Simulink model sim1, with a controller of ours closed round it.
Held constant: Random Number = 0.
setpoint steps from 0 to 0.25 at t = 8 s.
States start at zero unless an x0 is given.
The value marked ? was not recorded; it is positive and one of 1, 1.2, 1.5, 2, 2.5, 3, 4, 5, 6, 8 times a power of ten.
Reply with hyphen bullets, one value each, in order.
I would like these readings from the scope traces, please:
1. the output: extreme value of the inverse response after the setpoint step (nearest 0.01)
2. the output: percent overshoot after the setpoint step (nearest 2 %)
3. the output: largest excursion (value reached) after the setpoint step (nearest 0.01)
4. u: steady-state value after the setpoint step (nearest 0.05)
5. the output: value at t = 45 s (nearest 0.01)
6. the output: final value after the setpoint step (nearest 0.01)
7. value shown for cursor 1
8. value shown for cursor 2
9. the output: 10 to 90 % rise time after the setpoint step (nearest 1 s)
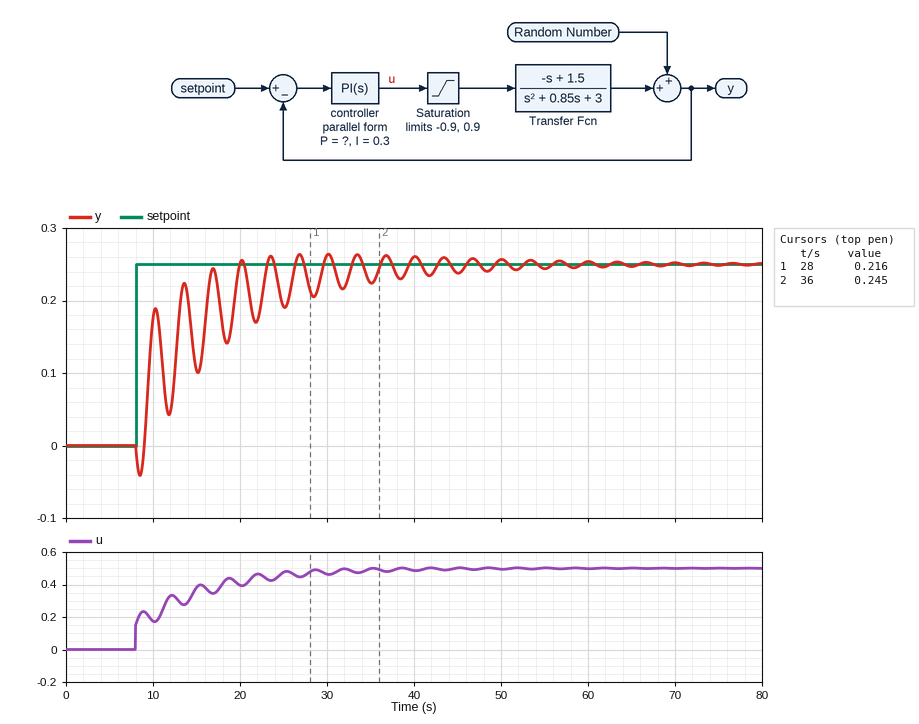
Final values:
- -0.04
- 6 %
- 0.26
- 0.50
- 0.24
- 0.25
- 0.216
- 0.245
- 7 s
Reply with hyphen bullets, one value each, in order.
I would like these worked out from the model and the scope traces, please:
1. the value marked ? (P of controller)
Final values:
- 0.6
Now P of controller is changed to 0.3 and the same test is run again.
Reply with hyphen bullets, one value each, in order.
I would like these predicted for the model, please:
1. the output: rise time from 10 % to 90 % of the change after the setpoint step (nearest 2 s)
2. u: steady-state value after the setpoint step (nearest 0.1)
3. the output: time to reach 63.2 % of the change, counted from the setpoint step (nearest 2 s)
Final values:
- 14 s
- 0.5
- 6 s
